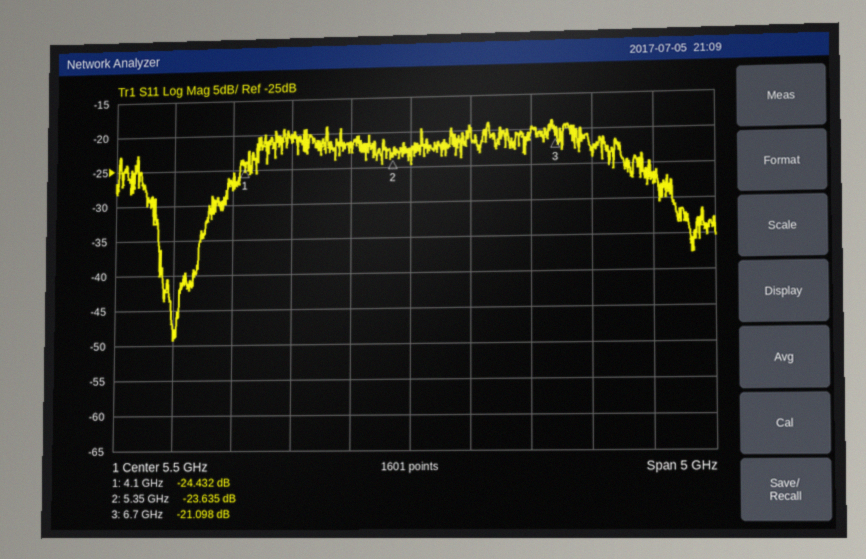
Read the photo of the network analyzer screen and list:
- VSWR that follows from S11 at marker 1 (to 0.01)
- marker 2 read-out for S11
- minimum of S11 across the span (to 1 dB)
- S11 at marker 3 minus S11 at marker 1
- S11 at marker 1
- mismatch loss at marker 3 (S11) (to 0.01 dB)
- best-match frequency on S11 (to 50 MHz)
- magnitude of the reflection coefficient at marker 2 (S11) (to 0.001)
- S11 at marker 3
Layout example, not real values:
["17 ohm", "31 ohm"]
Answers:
["1.13", "-23.635 dB", "-49 dB", "3.334 dB", "-24.432 dB", "0.03 dB", "3.50 GHz", "0.066", "-21.098 dB"]
